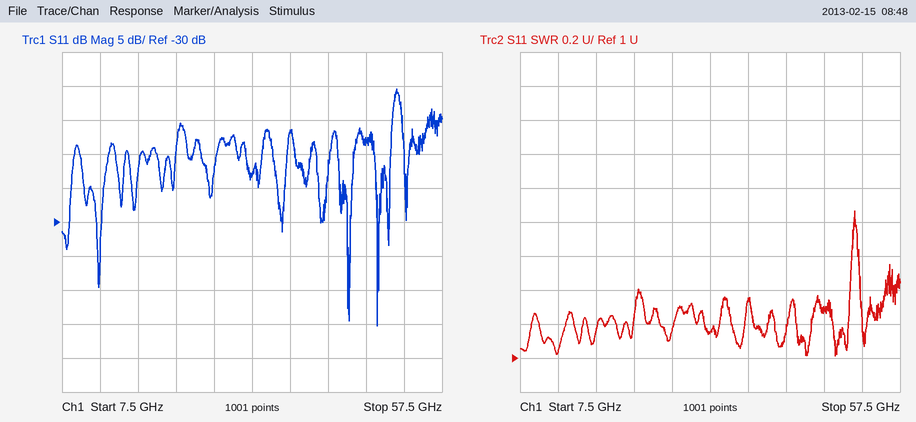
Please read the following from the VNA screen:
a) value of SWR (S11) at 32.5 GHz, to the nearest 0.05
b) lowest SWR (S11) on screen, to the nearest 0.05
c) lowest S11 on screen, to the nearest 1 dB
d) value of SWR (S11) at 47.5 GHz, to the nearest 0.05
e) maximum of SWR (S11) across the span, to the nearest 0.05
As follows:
1.15
1.00
-45 dB
1.30
1.85
